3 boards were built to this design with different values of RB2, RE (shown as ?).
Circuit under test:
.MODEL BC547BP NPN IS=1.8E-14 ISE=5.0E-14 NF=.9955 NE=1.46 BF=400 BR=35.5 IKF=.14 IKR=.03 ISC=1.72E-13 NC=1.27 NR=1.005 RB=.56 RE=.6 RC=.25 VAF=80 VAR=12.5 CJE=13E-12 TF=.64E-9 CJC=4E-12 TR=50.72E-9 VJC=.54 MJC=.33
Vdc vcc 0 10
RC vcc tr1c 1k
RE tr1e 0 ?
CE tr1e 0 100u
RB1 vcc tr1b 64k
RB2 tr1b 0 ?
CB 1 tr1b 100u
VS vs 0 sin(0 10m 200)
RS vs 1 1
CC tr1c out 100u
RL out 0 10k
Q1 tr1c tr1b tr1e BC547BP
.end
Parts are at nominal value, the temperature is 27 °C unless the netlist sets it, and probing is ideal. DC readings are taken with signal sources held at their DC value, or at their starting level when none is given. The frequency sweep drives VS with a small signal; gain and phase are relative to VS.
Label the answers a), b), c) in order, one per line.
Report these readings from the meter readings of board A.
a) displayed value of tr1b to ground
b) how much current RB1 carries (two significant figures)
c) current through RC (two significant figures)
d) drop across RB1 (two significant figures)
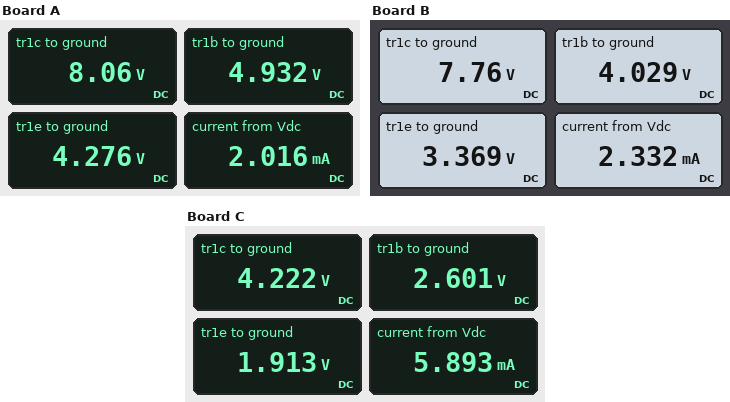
a) 4.932 V
b) 79 µA
c) 1.9 mA
d) 5.1 V
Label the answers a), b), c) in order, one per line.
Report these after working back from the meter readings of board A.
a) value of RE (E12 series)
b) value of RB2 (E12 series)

a) 2.2 kΩ
b) 68 kΩ
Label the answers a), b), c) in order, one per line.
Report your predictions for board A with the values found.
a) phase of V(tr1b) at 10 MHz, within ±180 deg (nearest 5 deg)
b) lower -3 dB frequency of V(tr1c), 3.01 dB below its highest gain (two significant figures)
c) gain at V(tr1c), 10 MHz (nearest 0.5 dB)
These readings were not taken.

a) 0 deg
b) 110 Hz
c) 36.0 dB
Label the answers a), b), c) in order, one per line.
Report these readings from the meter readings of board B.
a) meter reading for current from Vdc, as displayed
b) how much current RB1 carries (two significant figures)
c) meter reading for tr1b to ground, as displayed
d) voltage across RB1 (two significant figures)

a) 2.332 mA
b) 93 µA
c) 4.029 V
d) 6.0 V
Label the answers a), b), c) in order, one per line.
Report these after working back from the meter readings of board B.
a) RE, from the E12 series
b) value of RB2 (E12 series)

a) 1.5 kΩ
b) 47 kΩ
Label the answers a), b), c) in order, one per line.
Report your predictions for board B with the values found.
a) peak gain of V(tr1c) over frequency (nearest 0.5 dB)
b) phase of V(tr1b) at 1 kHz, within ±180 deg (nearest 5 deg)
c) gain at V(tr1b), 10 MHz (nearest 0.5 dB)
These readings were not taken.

a) 37.0 dB
b) 0 deg
c) 0 dB
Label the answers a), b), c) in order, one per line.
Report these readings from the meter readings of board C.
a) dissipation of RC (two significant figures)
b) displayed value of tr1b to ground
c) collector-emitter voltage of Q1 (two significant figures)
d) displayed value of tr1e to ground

a) 33 mW
b) 2.601 V
c) 2.3 V
d) 1.913 V
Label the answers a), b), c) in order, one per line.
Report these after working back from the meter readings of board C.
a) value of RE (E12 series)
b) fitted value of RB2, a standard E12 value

a) 330 Ω
b) 27 kΩ
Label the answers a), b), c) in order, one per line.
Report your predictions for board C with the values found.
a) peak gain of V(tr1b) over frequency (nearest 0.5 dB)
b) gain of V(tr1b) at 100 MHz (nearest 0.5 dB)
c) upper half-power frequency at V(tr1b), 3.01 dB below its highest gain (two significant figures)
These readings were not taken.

a) 0 dB
b) -1.0 dB
c) 690 MHz
